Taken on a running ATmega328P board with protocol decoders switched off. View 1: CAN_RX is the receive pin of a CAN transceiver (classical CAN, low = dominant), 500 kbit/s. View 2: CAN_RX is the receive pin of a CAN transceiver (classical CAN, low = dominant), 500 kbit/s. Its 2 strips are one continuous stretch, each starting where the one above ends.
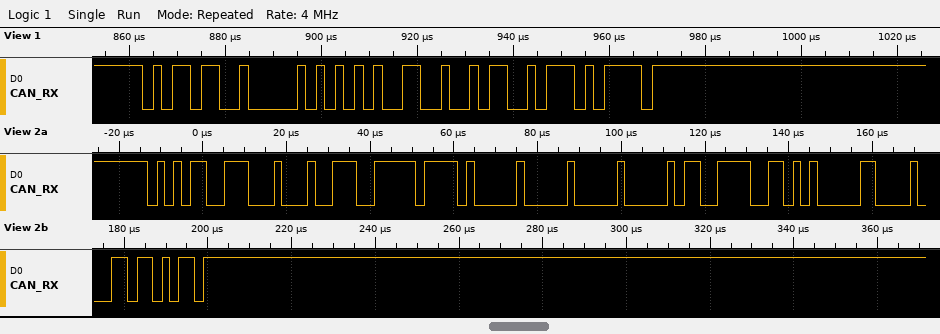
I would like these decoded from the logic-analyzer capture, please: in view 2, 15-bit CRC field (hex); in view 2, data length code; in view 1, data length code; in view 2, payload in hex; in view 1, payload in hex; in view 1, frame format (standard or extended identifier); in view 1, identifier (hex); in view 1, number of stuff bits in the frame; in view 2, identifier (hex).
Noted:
0x11B5
8
2
9C FF A0 00 00 CF 35 04
A9 92
standard
0x5B2
1
0x567
